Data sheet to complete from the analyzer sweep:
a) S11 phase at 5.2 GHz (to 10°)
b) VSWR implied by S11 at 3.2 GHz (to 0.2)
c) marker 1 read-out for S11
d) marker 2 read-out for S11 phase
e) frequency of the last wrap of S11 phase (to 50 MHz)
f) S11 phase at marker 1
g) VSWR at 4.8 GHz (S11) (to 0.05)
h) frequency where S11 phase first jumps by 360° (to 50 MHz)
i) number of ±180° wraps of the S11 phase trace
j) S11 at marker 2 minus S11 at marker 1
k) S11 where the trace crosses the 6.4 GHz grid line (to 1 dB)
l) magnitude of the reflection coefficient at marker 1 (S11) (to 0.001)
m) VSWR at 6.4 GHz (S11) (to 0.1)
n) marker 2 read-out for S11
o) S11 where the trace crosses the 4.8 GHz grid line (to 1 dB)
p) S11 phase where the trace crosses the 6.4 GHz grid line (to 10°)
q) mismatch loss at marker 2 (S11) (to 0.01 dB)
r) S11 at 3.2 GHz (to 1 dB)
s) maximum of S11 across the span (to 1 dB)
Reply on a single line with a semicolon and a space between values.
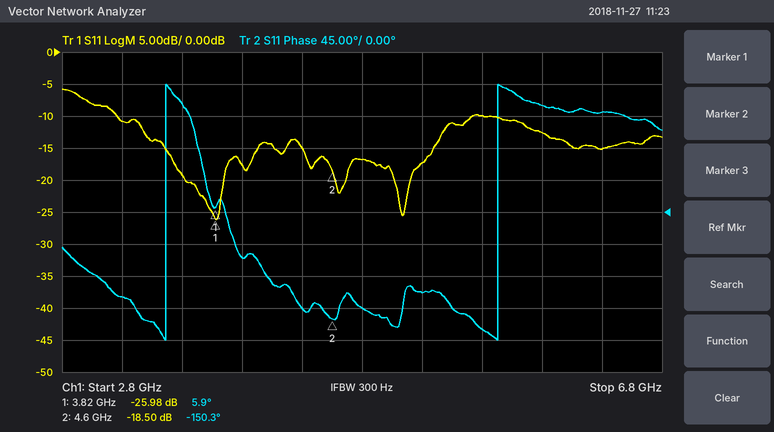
-110°; 1.8; -25.98 dB; -150.3°; 5.70 GHz; 5.9°; 1.35; 3.50 GHz; 2; 7.48 dB; -15 dB; 0.050; 1.4; -18.50 dB; -17 dB; 140°; 0.06 dB; -11 dB; -6 dB
